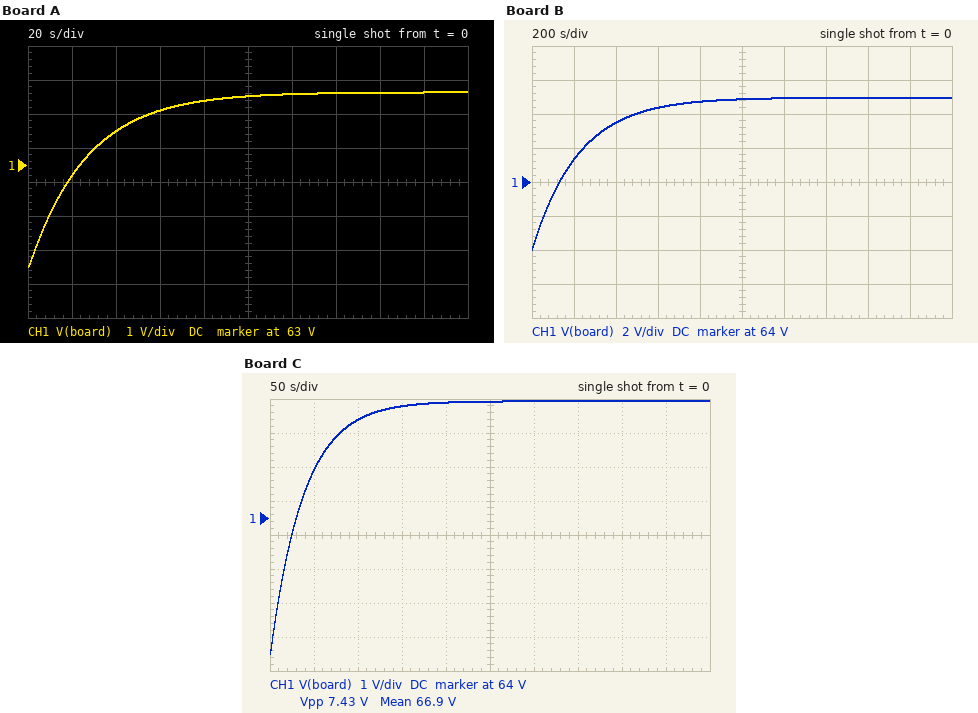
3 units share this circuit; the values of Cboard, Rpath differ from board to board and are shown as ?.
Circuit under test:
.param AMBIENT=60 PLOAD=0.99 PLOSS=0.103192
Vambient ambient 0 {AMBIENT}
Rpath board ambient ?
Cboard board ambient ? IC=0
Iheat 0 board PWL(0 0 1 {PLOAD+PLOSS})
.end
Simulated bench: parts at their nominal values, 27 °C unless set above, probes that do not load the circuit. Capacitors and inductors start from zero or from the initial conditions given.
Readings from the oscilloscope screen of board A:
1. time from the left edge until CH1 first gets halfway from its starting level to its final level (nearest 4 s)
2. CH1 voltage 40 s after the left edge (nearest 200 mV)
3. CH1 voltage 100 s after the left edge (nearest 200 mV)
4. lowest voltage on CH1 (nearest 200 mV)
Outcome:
20 s
64.0 V
65.0 V
60.0 V
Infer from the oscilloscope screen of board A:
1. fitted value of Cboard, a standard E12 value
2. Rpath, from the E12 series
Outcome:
5.6 F
4.7 Ω
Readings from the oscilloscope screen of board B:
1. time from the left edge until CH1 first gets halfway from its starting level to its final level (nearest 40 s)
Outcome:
160 s
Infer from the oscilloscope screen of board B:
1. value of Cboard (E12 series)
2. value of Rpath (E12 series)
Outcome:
27 F
8.2 Ω
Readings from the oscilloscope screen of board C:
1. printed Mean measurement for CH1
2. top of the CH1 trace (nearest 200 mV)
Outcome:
66.9 V
67.4 V
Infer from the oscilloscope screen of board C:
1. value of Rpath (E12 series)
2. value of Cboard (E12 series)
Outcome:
6.8 Ω
5.6 F
